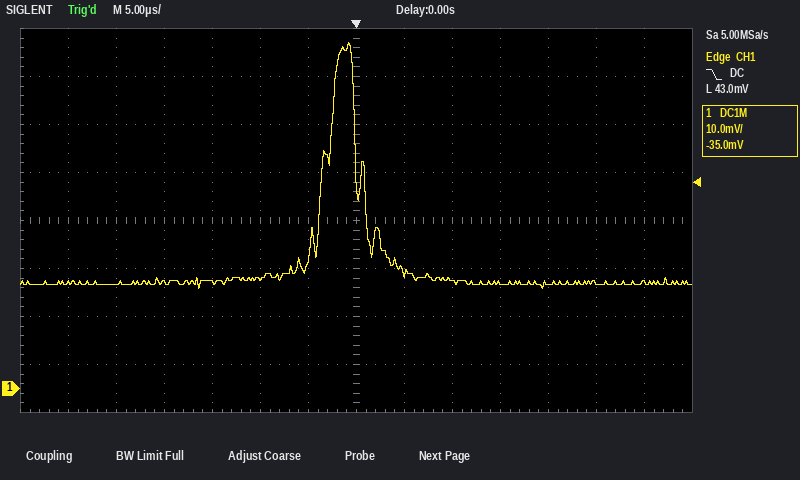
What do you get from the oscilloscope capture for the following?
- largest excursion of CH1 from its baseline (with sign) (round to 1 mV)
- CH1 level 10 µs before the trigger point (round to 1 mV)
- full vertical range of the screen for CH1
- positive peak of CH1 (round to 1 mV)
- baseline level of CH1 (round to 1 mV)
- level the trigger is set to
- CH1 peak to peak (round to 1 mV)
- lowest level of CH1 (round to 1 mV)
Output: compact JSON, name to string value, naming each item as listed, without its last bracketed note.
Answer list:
{"largest excursion of CH1 from its baseline (with sign)": "+50 mV", "CH1 level 10 µs before the trigger point": "23 mV", "full vertical range of the screen for CH1": "80 mV", "positive peak of CH1": "72 mV", "baseline level of CH1": "22 mV", "level the trigger is set to": "43.0 mV", "CH1 peak to peak": "51 mV", "lowest level of CH1": "21 mV"}
